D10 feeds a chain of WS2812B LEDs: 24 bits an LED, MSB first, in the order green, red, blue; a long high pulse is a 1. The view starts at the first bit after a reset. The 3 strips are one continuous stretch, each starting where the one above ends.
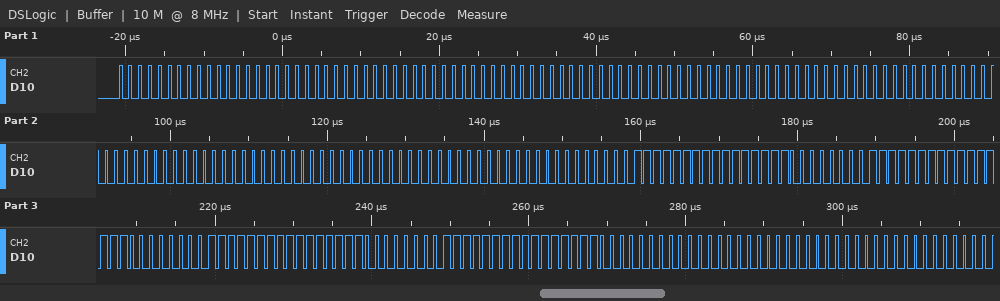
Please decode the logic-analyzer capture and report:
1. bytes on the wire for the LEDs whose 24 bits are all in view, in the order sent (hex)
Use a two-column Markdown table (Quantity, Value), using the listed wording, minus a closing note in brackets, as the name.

| Quantity | Value |
|---|---|
| bytes on the wire for the LEDs whose 24 bits are all in view, in the order sent | 00 00 00 00 00 00 00 00 00 00 00 00 00 00 00 00 00 00 FF FF 00 FF FF 00 FF FF 00 FF FF 00 00 00 00 |
